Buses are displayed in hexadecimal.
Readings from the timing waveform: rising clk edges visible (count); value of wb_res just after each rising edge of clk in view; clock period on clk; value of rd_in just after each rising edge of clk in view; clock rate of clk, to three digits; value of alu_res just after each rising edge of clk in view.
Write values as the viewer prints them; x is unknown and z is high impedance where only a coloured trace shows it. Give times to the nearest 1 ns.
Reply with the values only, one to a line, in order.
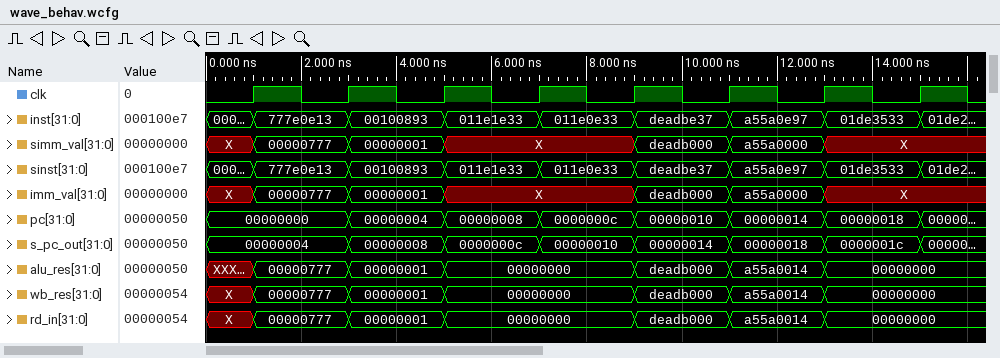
8
00000777, 00000001, 00000000, 00000000, deadb000, a55a0014, 00000000, 00000000
2 ns
00000777, 00000001, 00000000, 00000000, deadb000, a55a0014, 00000000, 00000000
500 MHz
00000777, 00000001, 00000000, 00000000, deadb000, a55a0014, 00000000, 00000000
